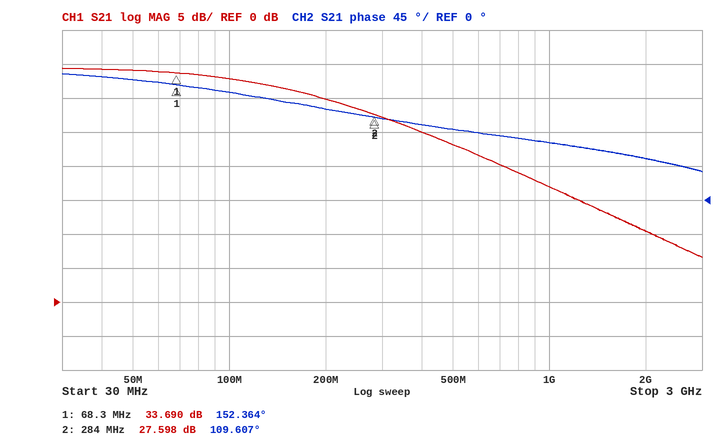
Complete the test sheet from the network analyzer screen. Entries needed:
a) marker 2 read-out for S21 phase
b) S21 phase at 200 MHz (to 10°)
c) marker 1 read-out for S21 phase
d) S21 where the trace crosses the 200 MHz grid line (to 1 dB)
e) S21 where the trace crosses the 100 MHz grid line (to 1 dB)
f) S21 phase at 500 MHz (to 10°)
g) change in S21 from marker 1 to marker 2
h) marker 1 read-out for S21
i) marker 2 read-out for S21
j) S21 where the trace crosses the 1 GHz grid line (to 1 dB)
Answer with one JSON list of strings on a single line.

["109.607°", "120°", "152.364°", "30 dB", "33 dB", "90°", "-6.092 dB", "33.690 dB", "27.598 dB", "17 dB"]
